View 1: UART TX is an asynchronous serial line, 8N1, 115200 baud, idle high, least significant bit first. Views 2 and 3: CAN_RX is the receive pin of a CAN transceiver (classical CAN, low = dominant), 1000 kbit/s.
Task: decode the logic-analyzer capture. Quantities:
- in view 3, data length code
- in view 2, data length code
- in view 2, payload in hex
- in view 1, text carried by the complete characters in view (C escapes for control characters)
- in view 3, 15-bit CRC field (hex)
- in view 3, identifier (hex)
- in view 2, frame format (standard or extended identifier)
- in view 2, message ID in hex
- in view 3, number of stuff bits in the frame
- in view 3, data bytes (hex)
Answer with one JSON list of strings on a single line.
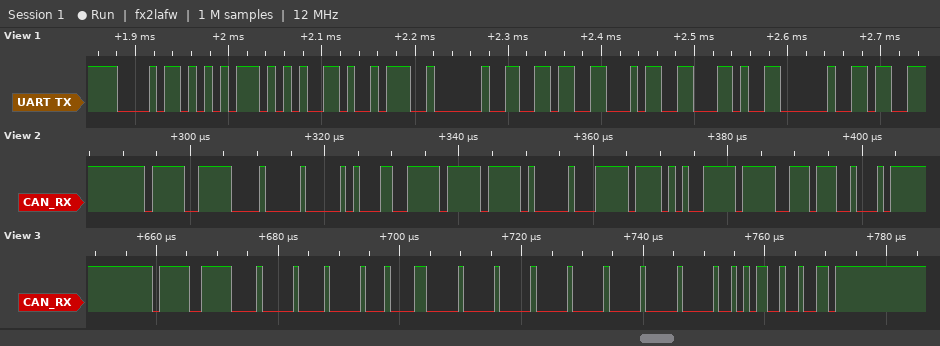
["8", "8", "00 8C FF FF 00 FF A9 FF", "\"hue: 64, \"", "0x5649", "0x7DF", "standard", "0x7DF", "12", "02 01 0C 00 00 00 00 00"]
